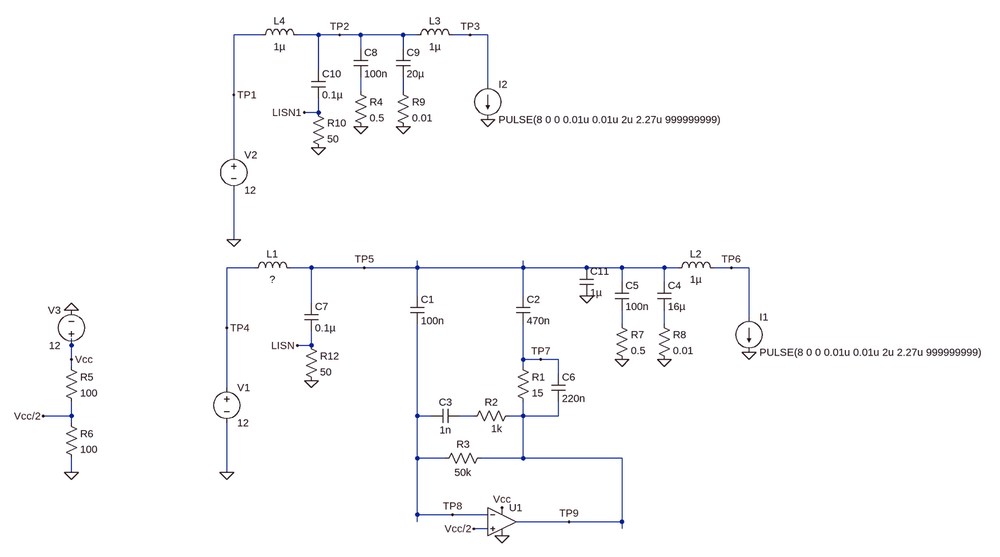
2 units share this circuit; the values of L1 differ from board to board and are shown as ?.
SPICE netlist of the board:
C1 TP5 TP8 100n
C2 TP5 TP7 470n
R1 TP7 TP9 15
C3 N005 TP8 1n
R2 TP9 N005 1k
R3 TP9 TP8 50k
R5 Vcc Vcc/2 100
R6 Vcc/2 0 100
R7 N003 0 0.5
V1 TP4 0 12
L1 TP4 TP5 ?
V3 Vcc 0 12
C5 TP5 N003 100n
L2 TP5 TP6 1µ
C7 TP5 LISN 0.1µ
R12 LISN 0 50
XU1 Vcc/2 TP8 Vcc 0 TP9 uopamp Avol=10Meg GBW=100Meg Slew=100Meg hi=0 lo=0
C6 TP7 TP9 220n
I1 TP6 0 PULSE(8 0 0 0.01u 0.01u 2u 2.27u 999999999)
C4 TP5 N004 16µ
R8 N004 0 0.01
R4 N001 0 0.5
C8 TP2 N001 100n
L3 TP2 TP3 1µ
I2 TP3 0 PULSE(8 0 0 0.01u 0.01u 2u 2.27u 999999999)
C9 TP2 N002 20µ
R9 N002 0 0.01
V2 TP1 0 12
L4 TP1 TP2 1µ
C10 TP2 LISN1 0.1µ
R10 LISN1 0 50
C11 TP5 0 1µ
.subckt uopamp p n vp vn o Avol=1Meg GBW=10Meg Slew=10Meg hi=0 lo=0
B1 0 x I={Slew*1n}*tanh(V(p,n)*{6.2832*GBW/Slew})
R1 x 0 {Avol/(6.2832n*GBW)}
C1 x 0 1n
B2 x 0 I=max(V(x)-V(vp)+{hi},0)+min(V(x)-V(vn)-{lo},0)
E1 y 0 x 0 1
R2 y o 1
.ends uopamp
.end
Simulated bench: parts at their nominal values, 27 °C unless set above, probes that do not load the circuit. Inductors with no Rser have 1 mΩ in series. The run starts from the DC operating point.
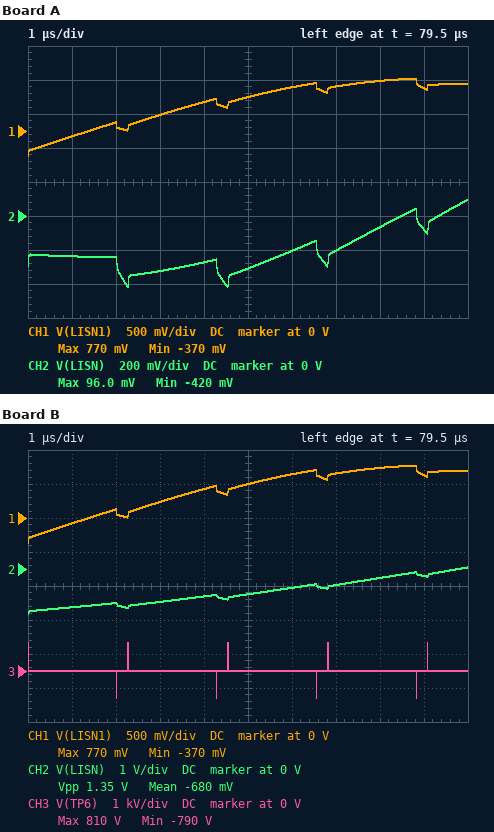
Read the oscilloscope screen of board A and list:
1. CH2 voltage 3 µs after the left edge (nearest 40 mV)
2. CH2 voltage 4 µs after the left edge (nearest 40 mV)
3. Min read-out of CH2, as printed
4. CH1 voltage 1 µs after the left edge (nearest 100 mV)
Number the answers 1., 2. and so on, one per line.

1. -320 mV
2. -280 mV
3. -420 mV
4. -100 mV
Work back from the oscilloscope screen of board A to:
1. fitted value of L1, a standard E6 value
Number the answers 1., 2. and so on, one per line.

1. 680 nH
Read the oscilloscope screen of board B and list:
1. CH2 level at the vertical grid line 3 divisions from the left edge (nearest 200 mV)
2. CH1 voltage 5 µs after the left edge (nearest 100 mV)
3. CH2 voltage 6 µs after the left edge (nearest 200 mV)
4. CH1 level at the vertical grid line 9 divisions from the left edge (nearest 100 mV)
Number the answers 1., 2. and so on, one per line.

1. -1.0 V
2. 500 mV
3. -600 mV
4. 600 mV
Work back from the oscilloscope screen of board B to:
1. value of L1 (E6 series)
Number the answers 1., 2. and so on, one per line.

1. 3.3 µH
